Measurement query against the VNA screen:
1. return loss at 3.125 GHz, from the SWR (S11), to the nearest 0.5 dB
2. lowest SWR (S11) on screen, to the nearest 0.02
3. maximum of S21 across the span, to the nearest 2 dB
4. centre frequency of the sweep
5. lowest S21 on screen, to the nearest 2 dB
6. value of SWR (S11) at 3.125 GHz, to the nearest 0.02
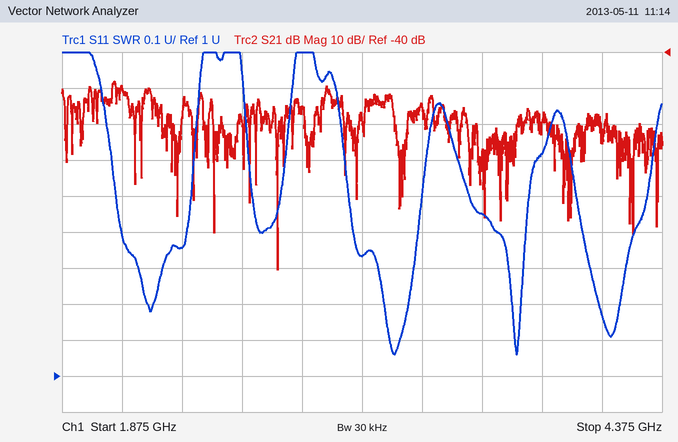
17.0 dB
1.06
-48 dB
3.125 GHz
-100 dB
1.34
